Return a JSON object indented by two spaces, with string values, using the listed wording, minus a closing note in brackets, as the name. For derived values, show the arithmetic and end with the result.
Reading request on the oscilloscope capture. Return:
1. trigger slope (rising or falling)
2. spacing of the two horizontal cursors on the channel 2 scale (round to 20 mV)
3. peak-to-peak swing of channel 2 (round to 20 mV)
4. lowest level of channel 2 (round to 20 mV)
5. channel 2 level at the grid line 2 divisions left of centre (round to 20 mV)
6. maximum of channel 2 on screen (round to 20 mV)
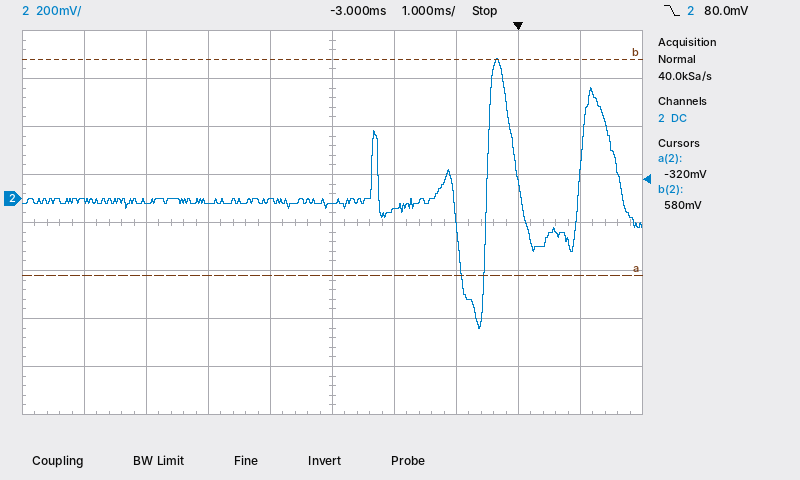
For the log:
{
  "trigger slope": "falling",
  "spacing of the two horizontal cursors on the channel 2 scale": "900 mV",
  "peak-to-peak swing of channel 2": "580 mV − (-540 mV) = 1.12 V",
  "lowest level of channel 2": "-540 mV",
  "channel 2 level at the grid line 2 divisions left of centre": "-20 mV",
  "maximum of channel 2 on screen": "580 mV"
}
